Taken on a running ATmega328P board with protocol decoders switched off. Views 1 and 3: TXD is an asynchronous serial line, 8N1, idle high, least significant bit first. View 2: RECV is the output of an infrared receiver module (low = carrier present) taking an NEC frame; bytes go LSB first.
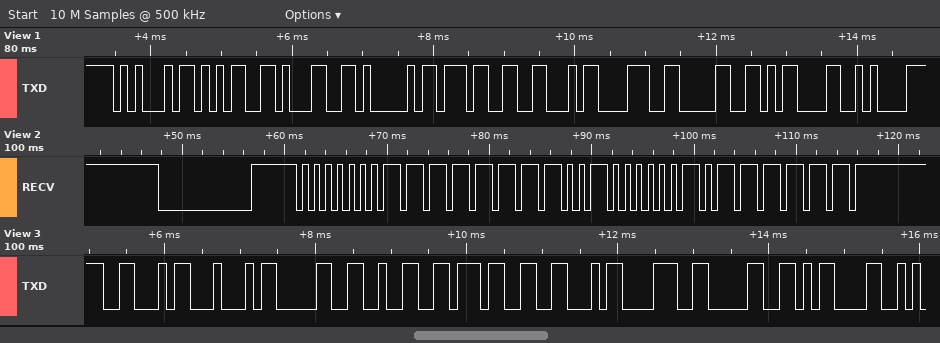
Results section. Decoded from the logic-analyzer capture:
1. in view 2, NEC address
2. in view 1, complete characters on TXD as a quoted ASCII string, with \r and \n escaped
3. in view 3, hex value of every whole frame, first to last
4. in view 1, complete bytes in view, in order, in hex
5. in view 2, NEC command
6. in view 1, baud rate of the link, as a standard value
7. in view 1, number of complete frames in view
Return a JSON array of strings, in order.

["0x80", "\"E51A7F80\\r\\n\"", "46 44 30 32 37 46 38 30 0D", "45 35 31 41 37 46 38 30 0D 0A", "0x02", "9600 baud", "10"]
